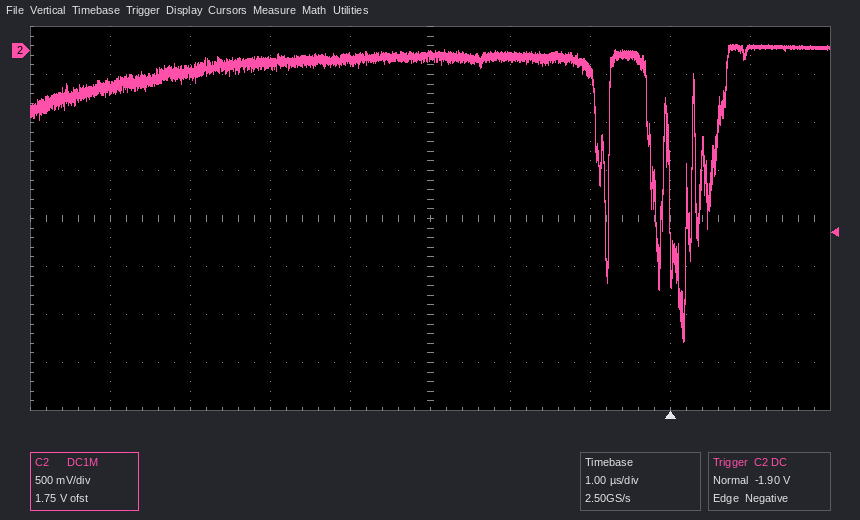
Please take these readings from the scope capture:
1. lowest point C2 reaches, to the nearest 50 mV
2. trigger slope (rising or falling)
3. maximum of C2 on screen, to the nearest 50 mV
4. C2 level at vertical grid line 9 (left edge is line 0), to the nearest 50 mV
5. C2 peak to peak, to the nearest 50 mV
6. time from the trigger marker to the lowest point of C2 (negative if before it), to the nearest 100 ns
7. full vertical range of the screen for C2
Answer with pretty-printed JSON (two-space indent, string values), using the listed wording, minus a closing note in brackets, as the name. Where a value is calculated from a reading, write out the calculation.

{
  "lowest point C2 reaches, to the nearest 50 mV": "-3.05 V",
  "trigger slope": "falling",
  "maximum of C2 on screen, to the nearest 50 mV": "50 mV",
  "C2 level at vertical grid line 9 (left edge is line 0), to the nearest 50 mV": "0 mV",
  "C2 peak to peak, to the nearest 50 mV": "50 mV − (-3.05 V) = 3.10 V",
  "time from the trigger marker to the lowest point of C2 (negative if before it), to the nearest 100 ns": "+200 ns",
  "full vertical range of the screen for C2": "4 V"
}
